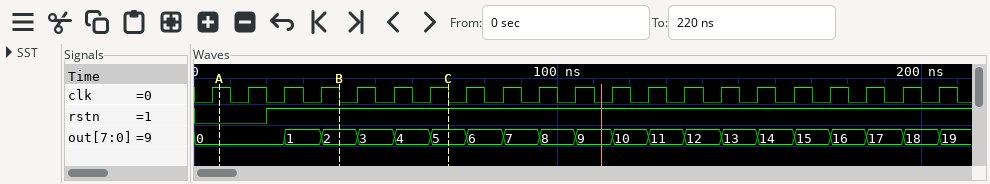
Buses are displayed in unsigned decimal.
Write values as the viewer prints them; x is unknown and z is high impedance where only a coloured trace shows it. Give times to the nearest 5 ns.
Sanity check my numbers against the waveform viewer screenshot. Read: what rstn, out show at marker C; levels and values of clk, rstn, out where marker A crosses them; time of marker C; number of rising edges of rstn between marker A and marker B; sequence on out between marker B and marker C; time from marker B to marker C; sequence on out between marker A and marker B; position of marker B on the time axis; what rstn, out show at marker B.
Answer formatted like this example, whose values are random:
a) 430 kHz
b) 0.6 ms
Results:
a) rstn=1, out=5
b) clk=1, rstn=0, out=0
c) 70 ns
d) 1
e) 2, 3, 4, 5
f) 30 ns
g) 0, 1, 2
h) 40 ns
i) rstn=1, out=2
